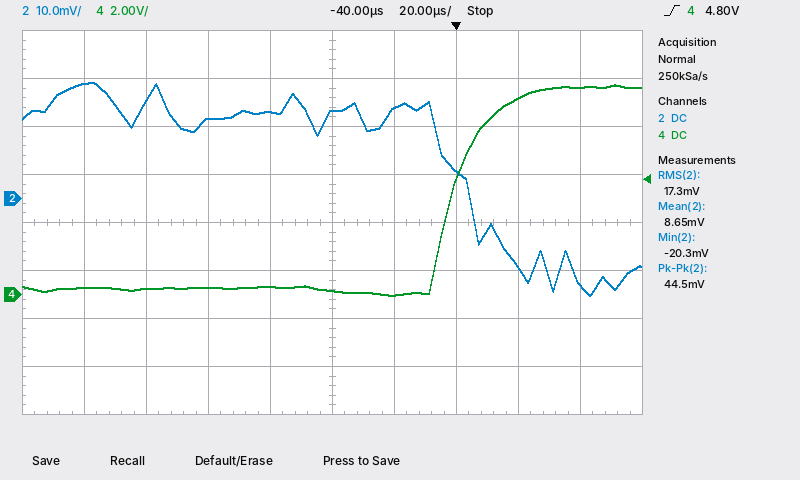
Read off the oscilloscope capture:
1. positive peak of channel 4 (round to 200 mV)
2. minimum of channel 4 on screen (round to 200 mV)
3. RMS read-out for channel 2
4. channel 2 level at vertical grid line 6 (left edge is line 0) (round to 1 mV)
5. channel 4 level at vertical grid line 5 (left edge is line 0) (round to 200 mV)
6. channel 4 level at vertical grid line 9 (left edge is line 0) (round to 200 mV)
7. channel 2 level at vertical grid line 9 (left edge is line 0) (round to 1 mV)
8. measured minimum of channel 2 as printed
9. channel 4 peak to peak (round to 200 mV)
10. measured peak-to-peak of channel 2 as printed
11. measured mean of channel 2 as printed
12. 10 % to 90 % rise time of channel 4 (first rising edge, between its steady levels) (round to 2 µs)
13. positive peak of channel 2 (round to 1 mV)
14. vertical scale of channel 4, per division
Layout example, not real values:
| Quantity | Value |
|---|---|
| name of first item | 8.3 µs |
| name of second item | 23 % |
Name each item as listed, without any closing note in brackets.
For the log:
| Quantity | Value |
|---|---|
| positive peak of channel 4 | 8.8 V |
| minimum of channel 4 on screen | 0.0 V |
| RMS read-out for channel 2 | 17.3 mV |
| channel 2 level at vertical grid line 6 (left edge is line 0) | 19 mV |
| channel 4 level at vertical grid line 5 (left edge is line 0) | 200 mV |
| channel 4 level at vertical grid line 9 (left edge is line 0) | 8.6 V |
| channel 2 level at vertical grid line 9 (left edge is line 0) | -18 mV |
| measured minimum of channel 2 as printed | -20.3 mV |
| channel 4 peak to peak | 8.8 V |
| measured peak-to-peak of channel 2 as printed | 44.5 mV |
| measured mean of channel 2 as printed | 8.65 mV |
| 10 % to 90 % rise time of channel 4 (first rising edge, between its steady levels) | 22 µs |
| positive peak of channel 2 | 24 mV |
| vertical scale of channel 4, per division | 2 V |
